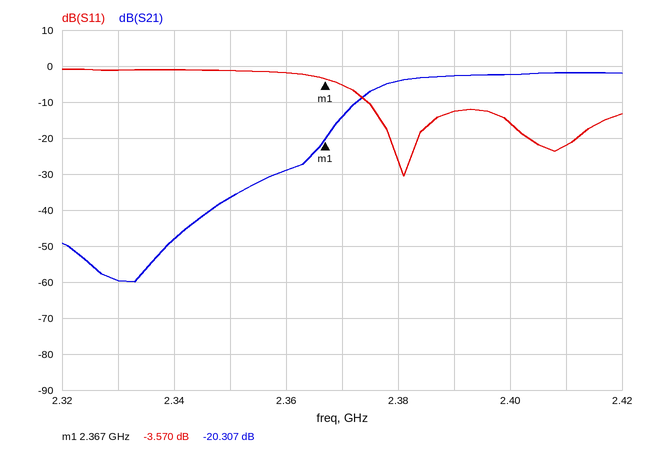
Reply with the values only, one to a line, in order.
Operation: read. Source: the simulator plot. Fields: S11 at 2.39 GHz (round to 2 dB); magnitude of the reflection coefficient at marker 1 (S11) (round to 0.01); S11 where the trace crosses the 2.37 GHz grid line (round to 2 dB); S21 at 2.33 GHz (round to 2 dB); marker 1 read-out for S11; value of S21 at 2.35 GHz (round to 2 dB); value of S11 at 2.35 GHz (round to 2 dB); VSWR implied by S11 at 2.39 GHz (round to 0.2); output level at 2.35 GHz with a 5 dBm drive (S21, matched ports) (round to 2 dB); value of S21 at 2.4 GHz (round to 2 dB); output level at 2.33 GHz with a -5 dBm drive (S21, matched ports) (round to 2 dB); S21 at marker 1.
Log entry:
-12 dB
0.66
-6 dB
-60 dB
-3.570 dB
-36 dB
-2 dB
1.6
-32 dBm
-2 dB
-64 dBm
-20.307 dB
